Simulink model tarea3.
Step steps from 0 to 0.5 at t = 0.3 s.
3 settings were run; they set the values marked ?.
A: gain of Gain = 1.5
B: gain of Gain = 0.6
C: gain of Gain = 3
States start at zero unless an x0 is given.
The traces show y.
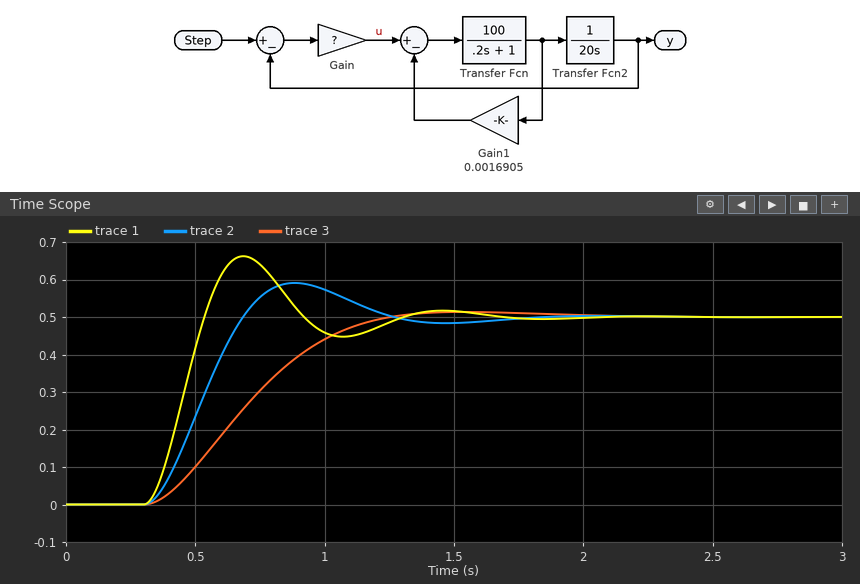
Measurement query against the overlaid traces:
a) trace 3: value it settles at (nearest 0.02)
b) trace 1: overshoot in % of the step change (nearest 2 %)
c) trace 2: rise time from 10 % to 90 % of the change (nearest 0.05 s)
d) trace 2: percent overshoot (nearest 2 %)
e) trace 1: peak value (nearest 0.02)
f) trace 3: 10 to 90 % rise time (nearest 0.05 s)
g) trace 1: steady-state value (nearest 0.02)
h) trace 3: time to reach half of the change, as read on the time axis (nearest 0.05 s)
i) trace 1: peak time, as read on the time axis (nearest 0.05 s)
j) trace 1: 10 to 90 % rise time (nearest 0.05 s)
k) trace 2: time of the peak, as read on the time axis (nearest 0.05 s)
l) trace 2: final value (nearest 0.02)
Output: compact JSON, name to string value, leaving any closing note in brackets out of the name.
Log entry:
{"trace 3: value it settles at": "0.50", "trace 1: overshoot in % of the step change": "32 %", "trace 2: rise time from 10 % to 90 % of the change": "0.25 s", "trace 2: percent overshoot": "18 %", "trace 1: peak value": "0.66", "trace 3: 10 to 90 % rise time": "0.60 s", "trace 1: steady-state value": "0.50", "trace 3: time to reach half of the change, as read on the time axis": "0.70 s", "trace 1: peak time, as read on the time axis": "0.70 s", "trace 1: 10 to 90 % rise time": "0.15 s", "trace 2: time of the peak, as read on the time axis": "0.90 s", "trace 2: final value": "0.50"}
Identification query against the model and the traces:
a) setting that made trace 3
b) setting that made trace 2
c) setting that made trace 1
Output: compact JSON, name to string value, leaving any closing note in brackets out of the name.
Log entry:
{"setting that made trace 3": "B", "setting that made trace 2": "A", "setting that made trace 1": "C"}
